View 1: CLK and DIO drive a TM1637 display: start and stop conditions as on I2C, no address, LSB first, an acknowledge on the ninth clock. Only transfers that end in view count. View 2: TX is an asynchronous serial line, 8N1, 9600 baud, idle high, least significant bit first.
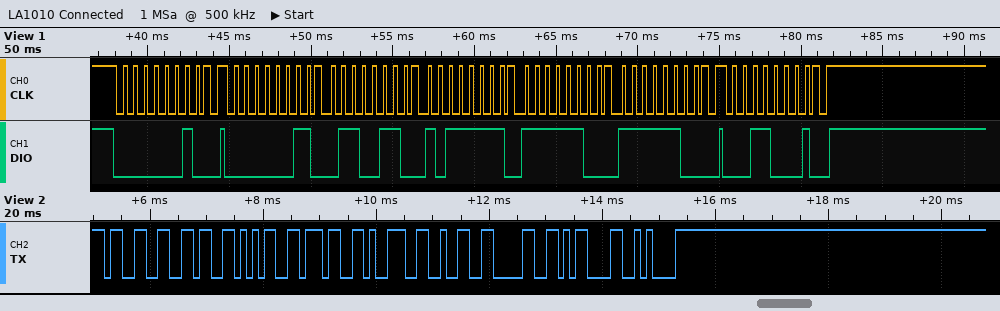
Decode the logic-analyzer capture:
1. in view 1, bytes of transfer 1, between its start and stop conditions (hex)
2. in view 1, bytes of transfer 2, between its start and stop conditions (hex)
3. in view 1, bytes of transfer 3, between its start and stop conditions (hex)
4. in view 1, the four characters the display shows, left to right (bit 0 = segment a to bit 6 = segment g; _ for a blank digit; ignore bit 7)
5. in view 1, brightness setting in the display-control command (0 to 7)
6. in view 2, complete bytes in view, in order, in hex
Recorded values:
40
C0 66 FD 3F 3F
8C
4600
4
33 36 35 37 39 32 30 0D 0A
